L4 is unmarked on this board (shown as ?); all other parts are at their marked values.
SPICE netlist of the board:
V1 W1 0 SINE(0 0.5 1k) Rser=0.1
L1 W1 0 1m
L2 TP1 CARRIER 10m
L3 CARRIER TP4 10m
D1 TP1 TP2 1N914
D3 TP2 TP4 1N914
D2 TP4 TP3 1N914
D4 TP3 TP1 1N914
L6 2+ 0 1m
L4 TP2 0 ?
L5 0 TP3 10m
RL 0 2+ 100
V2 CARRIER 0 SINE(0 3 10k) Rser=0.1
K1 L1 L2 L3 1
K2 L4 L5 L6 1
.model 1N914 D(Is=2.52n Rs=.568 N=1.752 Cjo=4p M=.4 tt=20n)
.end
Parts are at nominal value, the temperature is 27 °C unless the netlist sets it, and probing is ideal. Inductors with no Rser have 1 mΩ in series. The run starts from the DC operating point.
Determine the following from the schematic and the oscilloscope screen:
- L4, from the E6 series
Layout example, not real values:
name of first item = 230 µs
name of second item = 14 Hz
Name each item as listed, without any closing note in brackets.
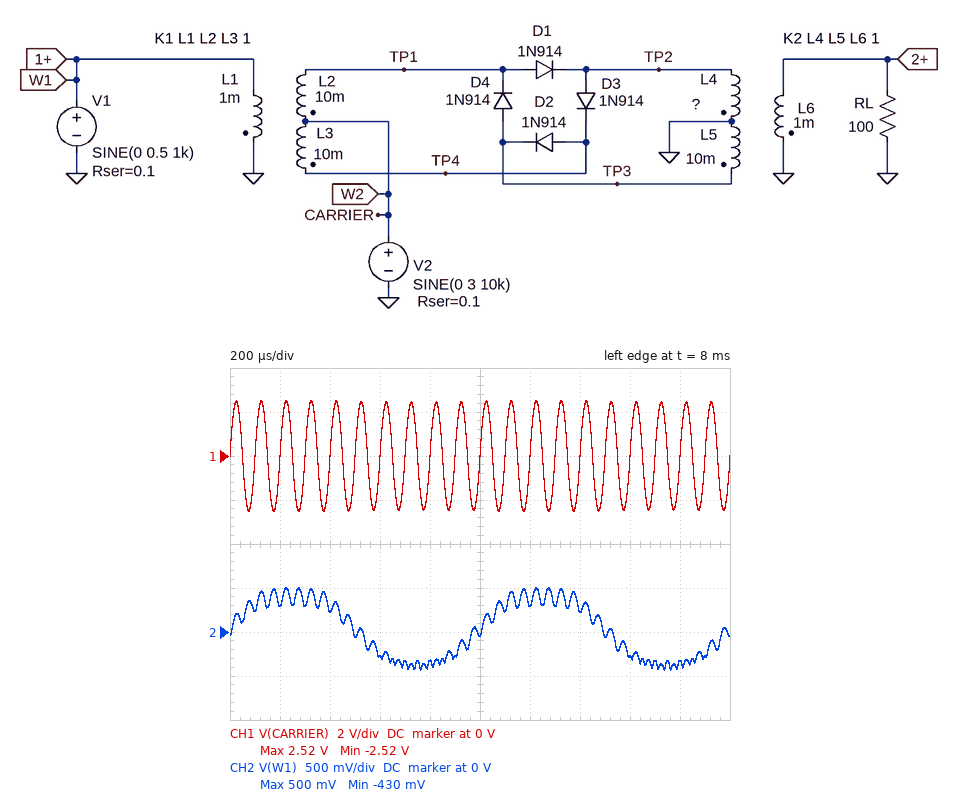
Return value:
L4, from the E6 series = 15 mH
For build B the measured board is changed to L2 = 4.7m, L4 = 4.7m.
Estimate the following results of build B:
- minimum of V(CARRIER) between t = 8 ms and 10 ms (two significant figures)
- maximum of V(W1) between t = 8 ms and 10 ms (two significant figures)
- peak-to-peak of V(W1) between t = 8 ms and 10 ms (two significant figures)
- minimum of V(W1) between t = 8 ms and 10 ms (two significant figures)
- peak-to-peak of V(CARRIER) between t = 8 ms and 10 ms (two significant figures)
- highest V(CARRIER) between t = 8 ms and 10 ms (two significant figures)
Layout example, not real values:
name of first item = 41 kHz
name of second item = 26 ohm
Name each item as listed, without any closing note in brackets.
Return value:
minimum of V(CARRIER) between t = 8 ms and 10 ms = -2.6 V
maximum of V(W1) between t = 8 ms and 10 ms = 510 mV
peak-to-peak of V(W1) between t = 8 ms and 10 ms = 1.1 V
minimum of V(W1) between t = 8 ms and 10 ms = -570 mV
peak-to-peak of V(CARRIER) between t = 8 ms and 10 ms = 5.1 V
highest V(CARRIER) between t = 8 ms and 10 ms = 2.5 V
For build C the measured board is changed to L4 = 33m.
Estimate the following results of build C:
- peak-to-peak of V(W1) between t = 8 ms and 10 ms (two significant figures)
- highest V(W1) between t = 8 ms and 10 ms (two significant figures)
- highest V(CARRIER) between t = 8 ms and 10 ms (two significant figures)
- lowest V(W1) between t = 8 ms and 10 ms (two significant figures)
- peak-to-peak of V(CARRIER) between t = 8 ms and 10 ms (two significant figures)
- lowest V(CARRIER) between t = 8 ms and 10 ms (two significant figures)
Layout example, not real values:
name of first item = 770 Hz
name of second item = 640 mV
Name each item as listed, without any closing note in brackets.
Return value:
peak-to-peak of V(W1) between t = 8 ms and 10 ms = 870 mV
highest V(W1) between t = 8 ms and 10 ms = 480 mV
highest V(CARRIER) between t = 8 ms and 10 ms = 2.6 V
lowest V(W1) between t = 8 ms and 10 ms = -390 mV
peak-to-peak of V(CARRIER) between t = 8 ms and 10 ms = 5.2 V
lowest V(CARRIER) between t = 8 ms and 10 ms = -2.6 V
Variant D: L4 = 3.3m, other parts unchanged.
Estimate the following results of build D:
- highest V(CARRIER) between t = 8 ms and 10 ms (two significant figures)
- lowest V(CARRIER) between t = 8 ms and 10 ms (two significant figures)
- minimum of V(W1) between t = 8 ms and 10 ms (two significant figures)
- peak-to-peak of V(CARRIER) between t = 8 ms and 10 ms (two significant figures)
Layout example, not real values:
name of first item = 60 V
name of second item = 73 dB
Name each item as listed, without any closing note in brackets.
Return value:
highest V(CARRIER) between t = 8 ms and 10 ms = 2.6 V
lowest V(CARRIER) between t = 8 ms and 10 ms = -2.6 V
minimum of V(W1) between t = 8 ms and 10 ms = -480 mV
peak-to-peak of V(CARRIER) between t = 8 ms and 10 ms = 5.2 V
